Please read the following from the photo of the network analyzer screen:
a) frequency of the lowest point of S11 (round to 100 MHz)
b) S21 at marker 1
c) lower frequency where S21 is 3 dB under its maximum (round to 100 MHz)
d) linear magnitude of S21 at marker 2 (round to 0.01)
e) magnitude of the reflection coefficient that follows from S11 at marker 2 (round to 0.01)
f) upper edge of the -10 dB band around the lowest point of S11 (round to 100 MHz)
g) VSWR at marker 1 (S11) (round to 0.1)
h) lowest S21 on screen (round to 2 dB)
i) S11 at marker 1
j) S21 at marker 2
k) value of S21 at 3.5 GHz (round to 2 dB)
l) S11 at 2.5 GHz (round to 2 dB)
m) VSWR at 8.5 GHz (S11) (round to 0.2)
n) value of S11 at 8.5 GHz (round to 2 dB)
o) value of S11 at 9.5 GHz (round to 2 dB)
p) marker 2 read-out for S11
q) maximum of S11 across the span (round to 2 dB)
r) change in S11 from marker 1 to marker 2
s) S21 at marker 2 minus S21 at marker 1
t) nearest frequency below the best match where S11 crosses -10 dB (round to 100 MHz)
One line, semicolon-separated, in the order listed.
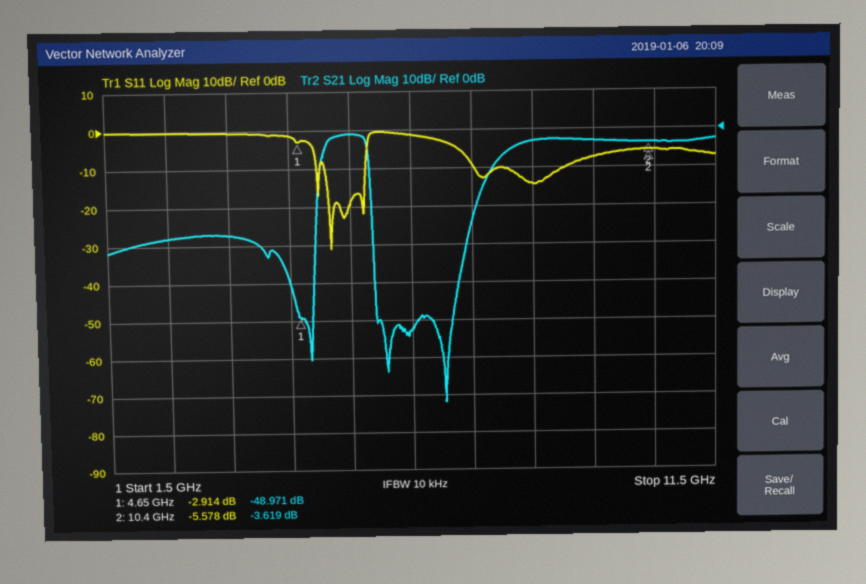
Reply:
5.2 GHz; -48.971 dB; 5.1 GHz; 0.66; 0.53; 5.8 GHz; 6.0; -72 dB; -2.914 dB; -3.619 dB; -28 dB; 0 dB; 1.4; -14 dB; -8 dB; -5.578 dB; 0 dB; -2.664 dB; 45.352 dB; 5.1 GHz
